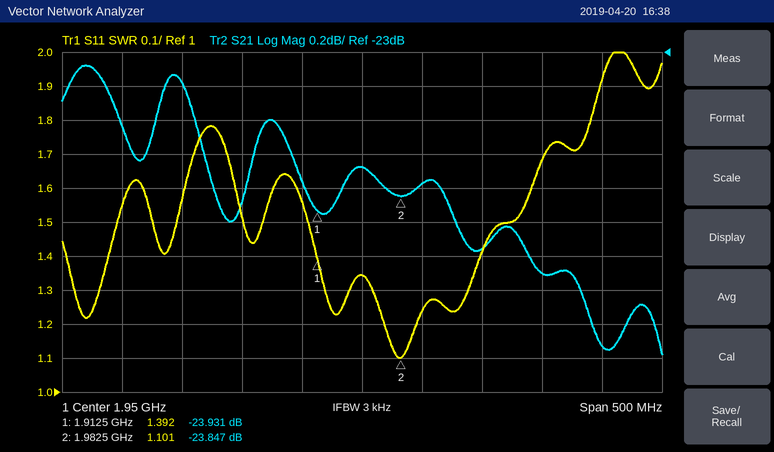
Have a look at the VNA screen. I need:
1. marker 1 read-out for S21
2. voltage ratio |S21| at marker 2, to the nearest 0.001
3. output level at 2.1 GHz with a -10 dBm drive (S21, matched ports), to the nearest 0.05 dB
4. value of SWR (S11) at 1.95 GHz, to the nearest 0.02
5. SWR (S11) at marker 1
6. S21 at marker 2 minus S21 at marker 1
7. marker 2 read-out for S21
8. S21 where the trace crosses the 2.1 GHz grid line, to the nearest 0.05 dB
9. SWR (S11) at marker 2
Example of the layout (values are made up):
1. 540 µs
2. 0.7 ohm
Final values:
1. -23.931 dB
2. 0.064
3. -34.30 dBm
4. 1.34
5. 1.392
6. 0.084 dB
7. -23.847 dB
8. -24.30 dB
9. 1.101
